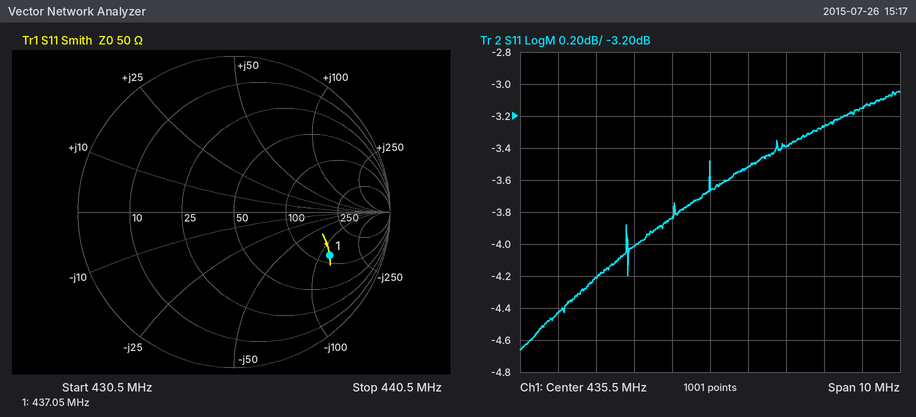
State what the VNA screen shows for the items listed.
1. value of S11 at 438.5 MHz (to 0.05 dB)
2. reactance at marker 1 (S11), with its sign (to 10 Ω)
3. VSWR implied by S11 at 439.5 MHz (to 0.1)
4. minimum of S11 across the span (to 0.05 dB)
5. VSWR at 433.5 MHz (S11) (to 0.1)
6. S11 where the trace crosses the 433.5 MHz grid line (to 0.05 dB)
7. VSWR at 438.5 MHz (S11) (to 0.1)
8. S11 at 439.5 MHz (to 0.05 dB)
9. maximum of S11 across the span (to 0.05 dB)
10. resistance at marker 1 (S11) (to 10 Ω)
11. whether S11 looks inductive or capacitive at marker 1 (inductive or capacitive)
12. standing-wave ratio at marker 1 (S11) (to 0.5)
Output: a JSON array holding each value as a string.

["-3.25 dB", "-120 Ω", "5.6", "-4.65 dB", "4.4", "-4.00 dB", "5.4", "-3.15 dB", "-3.05 dB", "120 Ω", "capacitive", "5.0"]
